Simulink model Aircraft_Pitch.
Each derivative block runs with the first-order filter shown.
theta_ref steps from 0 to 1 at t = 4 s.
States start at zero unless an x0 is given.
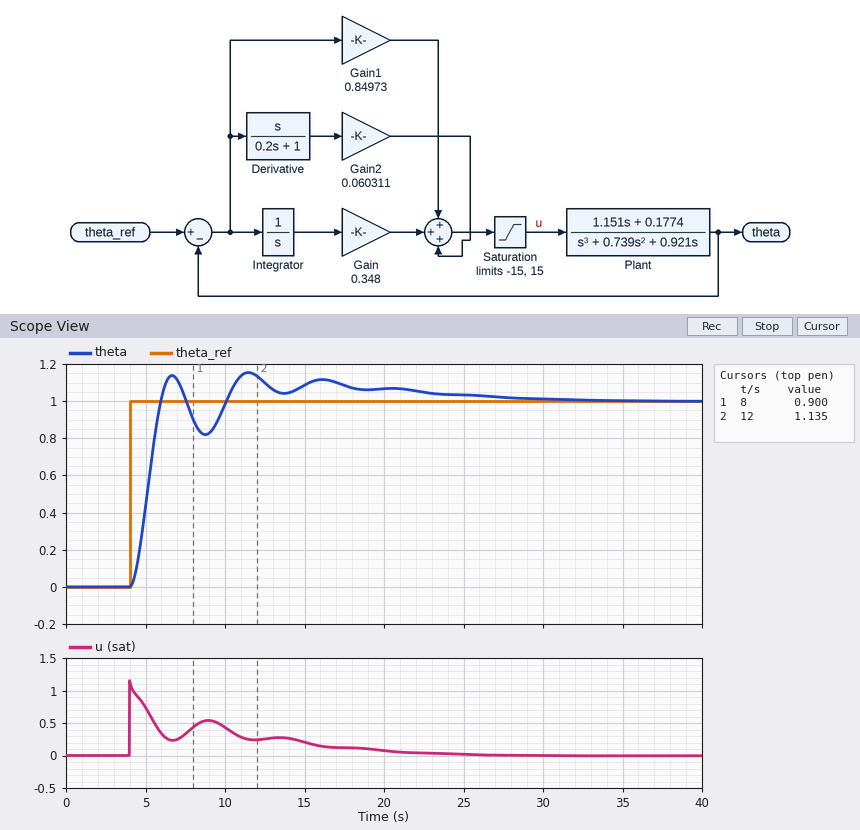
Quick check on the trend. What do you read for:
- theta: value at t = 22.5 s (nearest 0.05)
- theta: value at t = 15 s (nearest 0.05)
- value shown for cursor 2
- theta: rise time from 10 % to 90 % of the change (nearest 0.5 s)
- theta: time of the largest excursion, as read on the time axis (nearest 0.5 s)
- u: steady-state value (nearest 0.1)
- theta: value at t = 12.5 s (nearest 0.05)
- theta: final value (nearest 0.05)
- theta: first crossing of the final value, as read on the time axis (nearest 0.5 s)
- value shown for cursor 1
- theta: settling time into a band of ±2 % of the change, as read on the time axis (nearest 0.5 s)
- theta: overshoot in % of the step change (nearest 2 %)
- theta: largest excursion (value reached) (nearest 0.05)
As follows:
1.05
1.10
1.135
1.5 s
11.5 s
0.0
1.10
1.00
6.0 s
0.900
27.5 s
16 %
1.15
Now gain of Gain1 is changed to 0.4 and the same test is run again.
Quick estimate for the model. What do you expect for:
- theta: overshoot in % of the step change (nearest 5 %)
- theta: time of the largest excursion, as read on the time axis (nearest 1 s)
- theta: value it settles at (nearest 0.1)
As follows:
20 %
13 s
1.0
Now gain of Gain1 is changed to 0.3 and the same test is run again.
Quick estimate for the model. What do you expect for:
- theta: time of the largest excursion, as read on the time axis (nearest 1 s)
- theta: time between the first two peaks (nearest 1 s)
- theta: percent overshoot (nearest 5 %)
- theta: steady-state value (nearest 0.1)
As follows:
14 s
6 s
20 %
1.0
